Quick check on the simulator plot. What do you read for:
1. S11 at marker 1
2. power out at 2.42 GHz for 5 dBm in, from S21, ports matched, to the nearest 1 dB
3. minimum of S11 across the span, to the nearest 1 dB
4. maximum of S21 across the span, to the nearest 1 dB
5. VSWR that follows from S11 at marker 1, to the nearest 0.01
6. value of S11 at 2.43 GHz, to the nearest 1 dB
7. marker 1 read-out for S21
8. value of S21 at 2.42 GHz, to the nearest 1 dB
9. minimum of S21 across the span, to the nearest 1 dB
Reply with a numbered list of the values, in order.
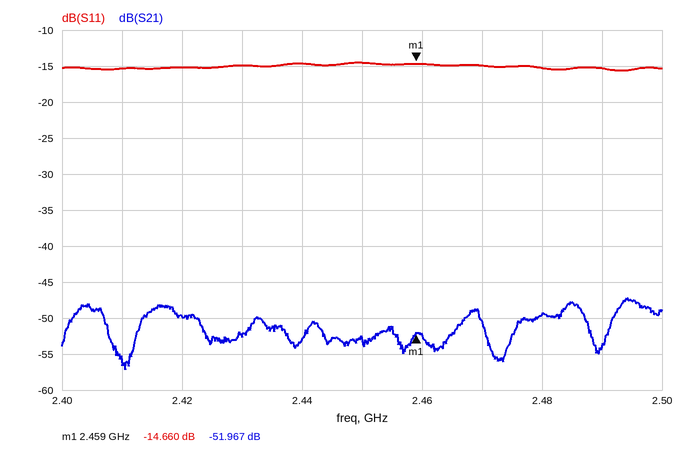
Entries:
1. -14.660 dB
2. -45 dBm
3. -16 dB
4. -47 dB
5. 1.45
6. -15 dB
7. -51.967 dB
8. -50 dB
9. -57 dB
